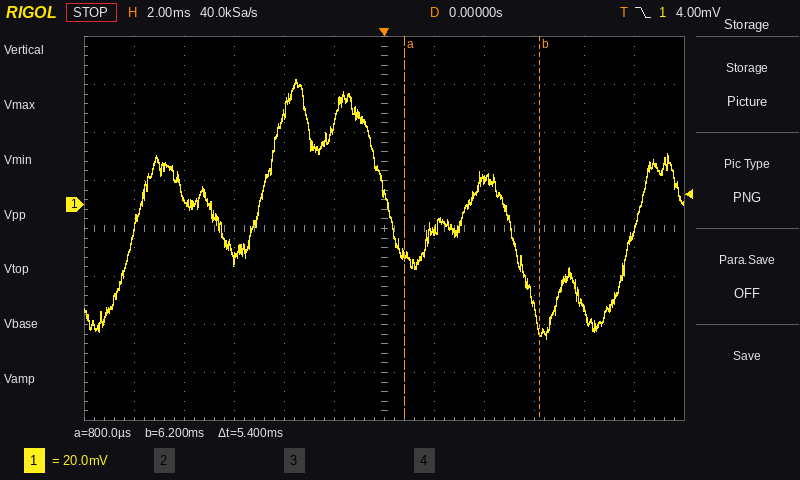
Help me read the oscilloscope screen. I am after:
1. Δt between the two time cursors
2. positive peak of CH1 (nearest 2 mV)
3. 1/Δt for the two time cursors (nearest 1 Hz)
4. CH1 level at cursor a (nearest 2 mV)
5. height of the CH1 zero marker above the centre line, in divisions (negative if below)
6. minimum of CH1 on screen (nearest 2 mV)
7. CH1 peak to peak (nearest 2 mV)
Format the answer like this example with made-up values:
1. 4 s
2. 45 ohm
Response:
1. 5.4 ms
2. 52 mV
3. 185 Hz
4. -20 mV
5. +0.5 div
6. -56 mV
7. 108 mV
